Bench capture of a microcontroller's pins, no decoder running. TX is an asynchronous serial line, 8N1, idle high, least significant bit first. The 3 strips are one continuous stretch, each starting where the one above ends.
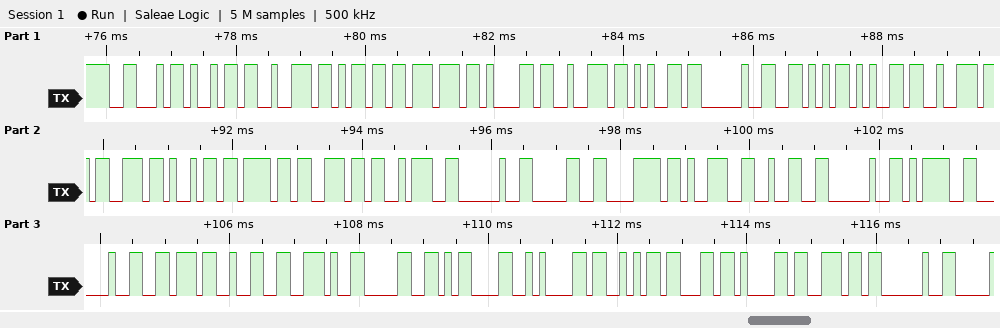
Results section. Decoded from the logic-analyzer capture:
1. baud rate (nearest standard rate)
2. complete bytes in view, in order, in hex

9600 baud
46 69 72 6D 77 61 72 65 20 56 65 72 73 69 6F 6E 3A 20 30 78 39 32 20 3D 20 76 32 2E 30 0D 0A 53 63 61 6E 20
